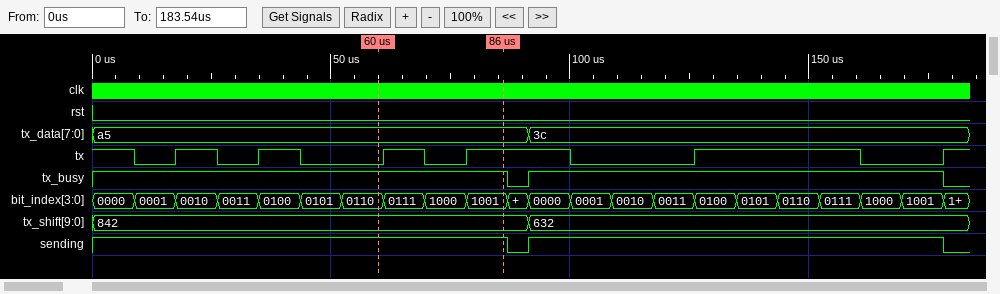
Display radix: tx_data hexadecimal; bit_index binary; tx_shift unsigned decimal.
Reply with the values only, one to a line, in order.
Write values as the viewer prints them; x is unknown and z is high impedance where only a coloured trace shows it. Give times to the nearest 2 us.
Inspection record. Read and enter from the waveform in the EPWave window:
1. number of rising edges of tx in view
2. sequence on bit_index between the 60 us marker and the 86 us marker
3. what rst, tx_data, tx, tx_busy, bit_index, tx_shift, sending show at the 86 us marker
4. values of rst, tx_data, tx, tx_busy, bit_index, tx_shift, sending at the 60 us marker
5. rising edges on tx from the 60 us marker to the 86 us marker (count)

6
0110, 0111, 1000, 1001
rst=0, tx_data=a5, tx=1, tx_busy=1, bit_index=1001, tx_shift=842, sending=1
rst=0, tx_data=a5, tx=0, tx_busy=1, bit_index=0110, tx_shift=842, sending=1
2
